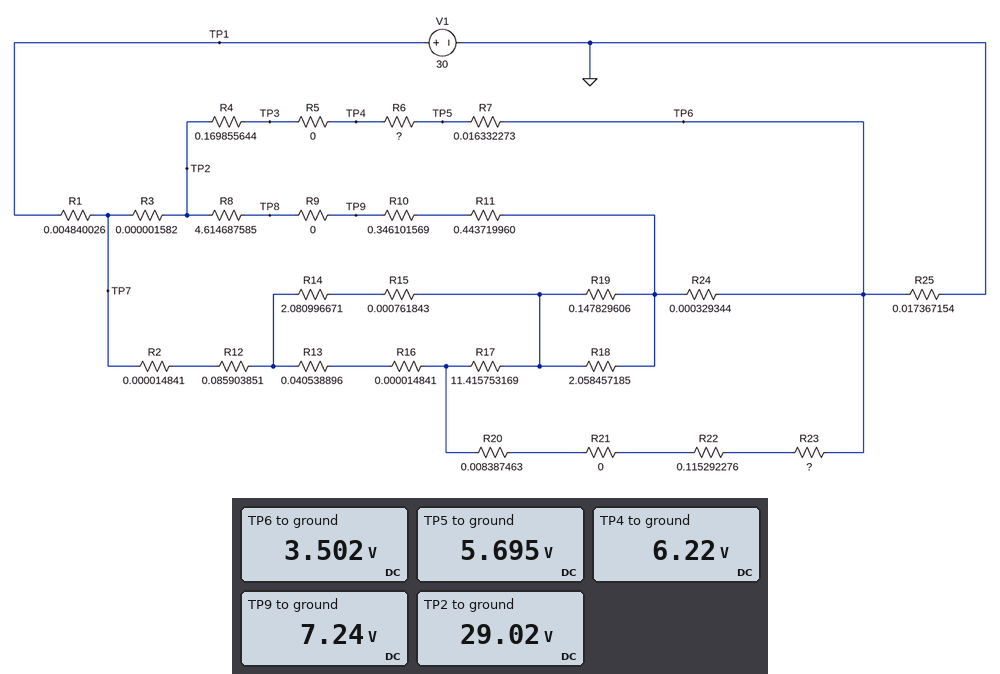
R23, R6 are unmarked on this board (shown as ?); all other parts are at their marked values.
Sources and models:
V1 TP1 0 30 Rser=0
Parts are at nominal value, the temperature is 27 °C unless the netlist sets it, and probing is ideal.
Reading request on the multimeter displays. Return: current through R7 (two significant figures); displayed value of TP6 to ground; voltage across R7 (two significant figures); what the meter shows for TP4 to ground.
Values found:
130 A
3.502 V
2.2 V
6.22 V
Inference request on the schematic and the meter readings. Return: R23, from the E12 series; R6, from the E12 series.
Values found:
0.22 Ω
3.9 mΩ
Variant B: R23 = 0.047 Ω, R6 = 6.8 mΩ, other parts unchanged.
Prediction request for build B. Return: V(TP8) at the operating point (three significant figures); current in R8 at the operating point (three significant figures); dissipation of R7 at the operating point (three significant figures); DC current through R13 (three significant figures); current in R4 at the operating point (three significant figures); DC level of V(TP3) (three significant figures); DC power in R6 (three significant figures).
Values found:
7.56 V
4.63 A
274 W
82.6 A
130 A
6.90 V
114 W
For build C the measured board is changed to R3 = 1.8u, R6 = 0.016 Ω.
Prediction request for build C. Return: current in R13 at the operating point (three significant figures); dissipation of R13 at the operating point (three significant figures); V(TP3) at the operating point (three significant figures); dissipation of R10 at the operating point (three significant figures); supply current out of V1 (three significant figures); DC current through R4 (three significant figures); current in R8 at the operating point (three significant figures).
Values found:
54.0 A
118 W
7.49 V
7.81 W
195 A
127 A
4.75 A
